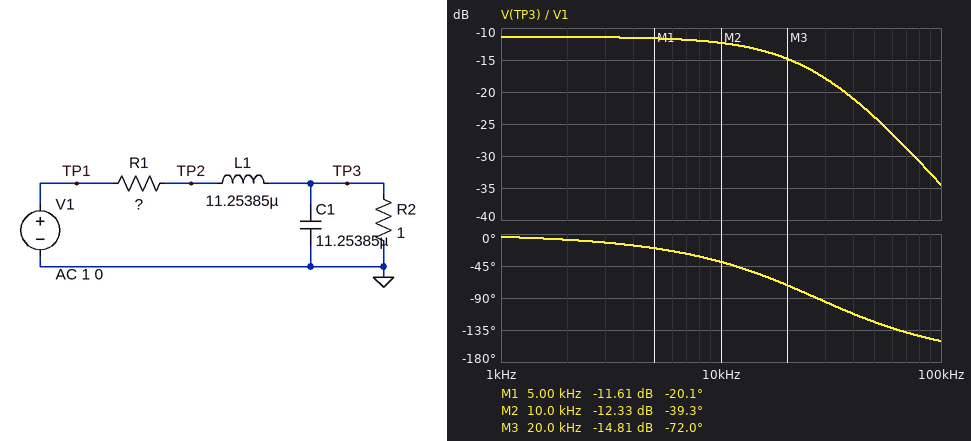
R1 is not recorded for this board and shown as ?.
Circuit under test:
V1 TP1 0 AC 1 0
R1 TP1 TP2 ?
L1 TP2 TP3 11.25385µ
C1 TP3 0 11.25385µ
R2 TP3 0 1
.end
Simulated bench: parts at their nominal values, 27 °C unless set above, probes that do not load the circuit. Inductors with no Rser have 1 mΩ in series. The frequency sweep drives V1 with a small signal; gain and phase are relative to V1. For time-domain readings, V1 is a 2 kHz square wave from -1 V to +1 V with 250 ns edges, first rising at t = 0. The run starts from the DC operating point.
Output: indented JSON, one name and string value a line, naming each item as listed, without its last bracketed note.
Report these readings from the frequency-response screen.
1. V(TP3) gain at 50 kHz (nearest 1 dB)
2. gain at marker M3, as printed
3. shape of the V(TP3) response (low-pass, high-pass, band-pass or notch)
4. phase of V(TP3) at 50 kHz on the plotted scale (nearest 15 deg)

{
  "V(TP3) gain at 50 kHz": "-24 dB",
  "gain at marker M3, as printed": "-14.81 dB",
  "shape of the V(TP3) response": "low-pass",
  "phase of V(TP3) at 50 kHz on the plotted scale": "-120 deg"
}
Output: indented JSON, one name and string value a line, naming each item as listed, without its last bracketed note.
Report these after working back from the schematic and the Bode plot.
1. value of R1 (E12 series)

{
  "value of R1": "2.7 Ω"
}
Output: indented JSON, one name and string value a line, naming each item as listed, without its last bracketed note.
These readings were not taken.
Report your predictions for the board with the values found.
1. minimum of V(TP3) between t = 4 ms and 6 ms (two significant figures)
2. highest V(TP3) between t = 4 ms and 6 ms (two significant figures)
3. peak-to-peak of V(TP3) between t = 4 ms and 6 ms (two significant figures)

{
  "minimum of V(TP3) between t = 4 ms and 6 ms": "-270 mV",
  "highest V(TP3) between t = 4 ms and 6 ms": "270 mV",
  "peak-to-peak of V(TP3) between t = 4 ms and 6 ms": "540 mV"
}
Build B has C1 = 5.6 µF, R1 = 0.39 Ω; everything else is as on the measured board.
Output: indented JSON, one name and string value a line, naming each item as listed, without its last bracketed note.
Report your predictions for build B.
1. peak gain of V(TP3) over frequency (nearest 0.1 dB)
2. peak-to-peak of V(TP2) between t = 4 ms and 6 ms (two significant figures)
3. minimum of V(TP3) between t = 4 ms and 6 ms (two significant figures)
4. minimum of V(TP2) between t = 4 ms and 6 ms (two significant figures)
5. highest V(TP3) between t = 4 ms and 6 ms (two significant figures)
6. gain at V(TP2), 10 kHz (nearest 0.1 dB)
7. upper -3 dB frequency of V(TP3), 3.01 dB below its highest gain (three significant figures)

{
  "peak gain of V(TP3) over frequency": "-2.9 dB",
  "peak-to-peak of V(TP2) between t = 4 ms and 6 ms": "2.5 V",
  "minimum of V(TP3) between t = 4 ms and 6 ms": "-780 mV",
  "minimum of V(TP2) between t = 4 ms and 6 ms": "-1.3 V",
  "highest V(TP3) between t = 4 ms and 6 ms": "780 mV",
  "gain at V(TP2), 10 kHz": "-2.8 dB",
  "upper -3 dB frequency of V(TP3), 3.01 dB below its highest gain": "23.3 kHz"
}
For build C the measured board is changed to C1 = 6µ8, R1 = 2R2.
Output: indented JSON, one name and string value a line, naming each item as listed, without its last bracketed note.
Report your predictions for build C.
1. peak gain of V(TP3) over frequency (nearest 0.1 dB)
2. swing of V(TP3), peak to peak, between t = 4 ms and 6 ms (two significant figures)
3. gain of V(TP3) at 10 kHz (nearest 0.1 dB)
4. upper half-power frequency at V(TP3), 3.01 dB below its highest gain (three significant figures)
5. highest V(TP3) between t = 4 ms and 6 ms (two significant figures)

{
  "peak gain of V(TP3) over frequency": "-10.1 dB",
  "swing of V(TP3), peak to peak, between t = 4 ms and 6 ms": "640 mV",
  "gain of V(TP3) at 10 kHz": "-10.5 dB",
  "upper half-power frequency at V(TP3), 3.01 dB below its highest gain": "26.7 kHz",
  "highest V(TP3) between t = 4 ms and 6 ms": "320 mV"
}
